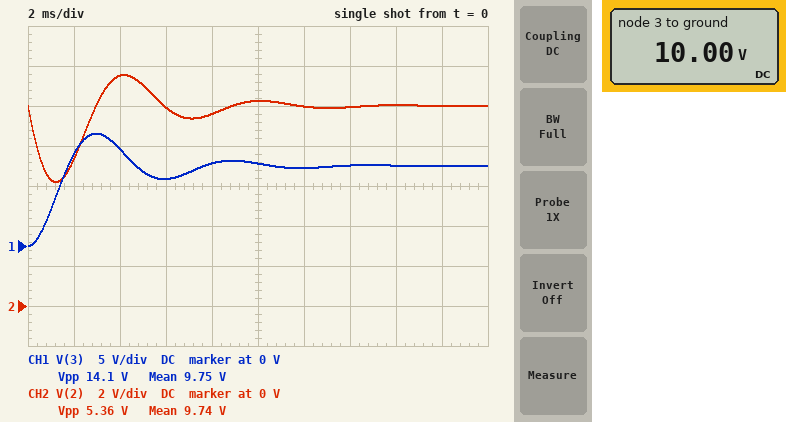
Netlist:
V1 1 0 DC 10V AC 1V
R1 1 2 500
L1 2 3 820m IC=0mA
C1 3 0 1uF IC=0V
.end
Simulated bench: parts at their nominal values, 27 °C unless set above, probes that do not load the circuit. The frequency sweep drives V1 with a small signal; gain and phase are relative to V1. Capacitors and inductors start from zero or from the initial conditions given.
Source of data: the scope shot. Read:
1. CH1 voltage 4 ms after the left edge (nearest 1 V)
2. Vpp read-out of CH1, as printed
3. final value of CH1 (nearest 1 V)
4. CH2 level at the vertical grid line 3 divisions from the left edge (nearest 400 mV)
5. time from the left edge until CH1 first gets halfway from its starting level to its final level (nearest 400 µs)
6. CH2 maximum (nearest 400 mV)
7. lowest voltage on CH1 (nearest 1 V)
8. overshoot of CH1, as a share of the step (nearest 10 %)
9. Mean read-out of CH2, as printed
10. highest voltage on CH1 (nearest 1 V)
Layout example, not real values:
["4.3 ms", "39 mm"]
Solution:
["12 V", "14.1 V", "10 V", "10.0 V", "1.2 ms", "11.6 V", "0 V", "40 %", "9.74 V", "14 V"]
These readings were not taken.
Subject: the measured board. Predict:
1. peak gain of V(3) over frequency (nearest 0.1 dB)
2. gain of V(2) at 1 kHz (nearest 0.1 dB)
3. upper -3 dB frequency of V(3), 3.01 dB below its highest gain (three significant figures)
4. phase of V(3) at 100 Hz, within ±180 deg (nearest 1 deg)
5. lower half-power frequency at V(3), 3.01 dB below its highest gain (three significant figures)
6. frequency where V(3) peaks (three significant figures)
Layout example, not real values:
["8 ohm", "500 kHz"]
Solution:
["5.5 dB", "0 dB", "206 Hz", "-25 deg", "98.9 Hz", "162 Hz"]
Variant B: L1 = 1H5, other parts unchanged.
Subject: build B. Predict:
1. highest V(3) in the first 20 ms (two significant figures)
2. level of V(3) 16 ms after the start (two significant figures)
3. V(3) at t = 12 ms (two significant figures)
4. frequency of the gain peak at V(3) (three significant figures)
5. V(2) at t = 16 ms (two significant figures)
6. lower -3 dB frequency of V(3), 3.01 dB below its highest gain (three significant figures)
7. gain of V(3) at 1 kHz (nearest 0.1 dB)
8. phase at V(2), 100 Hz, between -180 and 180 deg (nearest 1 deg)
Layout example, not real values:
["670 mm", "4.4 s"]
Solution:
["15 V", "9.3 V", "11 V", "124 Hz", "9.9 V", "93.4 Hz", "-35.3 dB", "-38 deg"]
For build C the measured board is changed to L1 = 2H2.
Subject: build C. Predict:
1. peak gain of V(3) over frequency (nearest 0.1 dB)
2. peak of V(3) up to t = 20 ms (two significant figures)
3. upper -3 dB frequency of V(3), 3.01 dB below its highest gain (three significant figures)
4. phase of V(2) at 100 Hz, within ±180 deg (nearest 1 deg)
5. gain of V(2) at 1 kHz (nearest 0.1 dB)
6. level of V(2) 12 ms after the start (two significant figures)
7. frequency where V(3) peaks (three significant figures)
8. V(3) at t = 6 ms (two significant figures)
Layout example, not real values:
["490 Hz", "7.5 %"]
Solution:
["9.6 dB", "16 V", "121 Hz", "-67 deg", "0 dB", "9.1 V", "104 Hz", "14 V"]
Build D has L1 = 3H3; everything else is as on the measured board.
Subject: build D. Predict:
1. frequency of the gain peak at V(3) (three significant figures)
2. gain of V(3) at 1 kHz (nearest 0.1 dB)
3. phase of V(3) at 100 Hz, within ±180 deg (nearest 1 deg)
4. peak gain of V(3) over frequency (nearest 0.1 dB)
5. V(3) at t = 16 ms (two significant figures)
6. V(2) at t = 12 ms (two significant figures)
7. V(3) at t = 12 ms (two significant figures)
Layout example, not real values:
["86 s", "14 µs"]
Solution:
["85.9 Hz", "-42.2 dB", "-134 deg", "11.3 dB", "12 V", "9.7 V", "6.0 V"]
